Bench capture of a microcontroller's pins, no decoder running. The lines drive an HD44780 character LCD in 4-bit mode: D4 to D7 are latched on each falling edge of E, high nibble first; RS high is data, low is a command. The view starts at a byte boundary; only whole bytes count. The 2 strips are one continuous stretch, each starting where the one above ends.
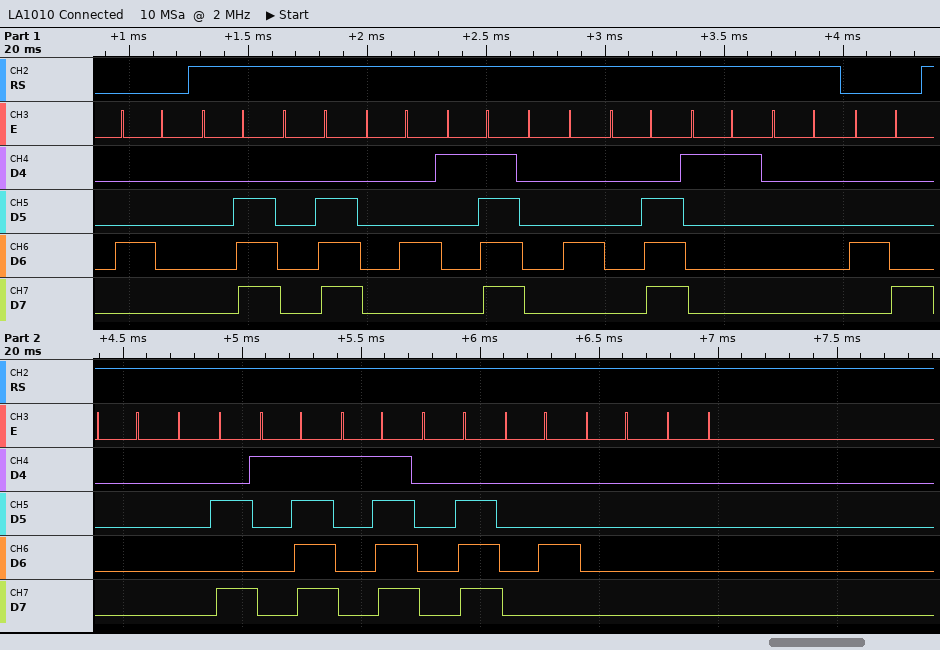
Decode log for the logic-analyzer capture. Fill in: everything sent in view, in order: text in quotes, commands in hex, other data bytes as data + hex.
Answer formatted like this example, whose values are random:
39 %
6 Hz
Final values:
0x40 data 0E 0E 04 1F 04 0E 11 00 0x48 data 00 0A 1F 1F 0E 04 00 00
